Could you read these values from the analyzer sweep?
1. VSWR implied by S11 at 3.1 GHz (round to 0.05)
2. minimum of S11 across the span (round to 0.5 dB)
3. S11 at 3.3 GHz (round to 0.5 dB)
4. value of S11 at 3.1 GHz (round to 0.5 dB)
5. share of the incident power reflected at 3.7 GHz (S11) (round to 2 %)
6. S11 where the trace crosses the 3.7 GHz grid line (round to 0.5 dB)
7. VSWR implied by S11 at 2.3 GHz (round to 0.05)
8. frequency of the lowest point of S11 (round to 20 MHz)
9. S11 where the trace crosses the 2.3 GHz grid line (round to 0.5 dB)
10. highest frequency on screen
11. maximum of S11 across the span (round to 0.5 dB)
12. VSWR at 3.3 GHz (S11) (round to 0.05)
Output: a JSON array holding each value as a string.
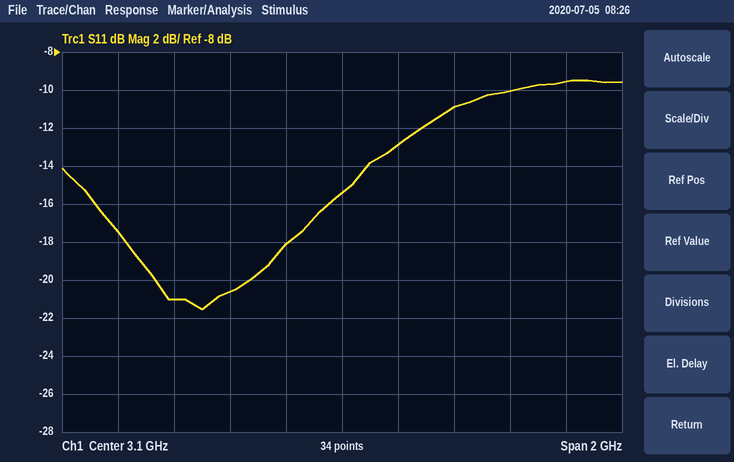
["1.40", "-21.5 dB", "-13.0 dB", "-15.5 dB", "10 %", "-10.0 dB", "1.30", "2.60 GHz", "-17.5 dB", "4.1 GHz", "-9.5 dB", "1.60"]
